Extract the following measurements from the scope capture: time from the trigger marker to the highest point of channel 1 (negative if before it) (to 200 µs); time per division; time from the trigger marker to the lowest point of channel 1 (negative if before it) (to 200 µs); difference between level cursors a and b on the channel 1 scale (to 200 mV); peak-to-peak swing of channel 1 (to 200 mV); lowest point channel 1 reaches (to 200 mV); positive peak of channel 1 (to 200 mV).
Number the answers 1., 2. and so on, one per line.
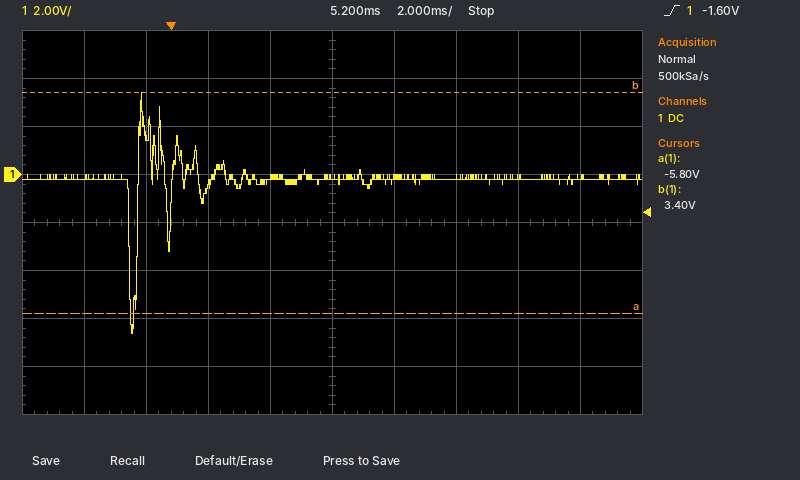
1. -1.0 ms
2. 2 ms
3. -1.2 ms
4. 9.2 V
5. 10.0 V
6. -6.6 V
7. 3.4 V
